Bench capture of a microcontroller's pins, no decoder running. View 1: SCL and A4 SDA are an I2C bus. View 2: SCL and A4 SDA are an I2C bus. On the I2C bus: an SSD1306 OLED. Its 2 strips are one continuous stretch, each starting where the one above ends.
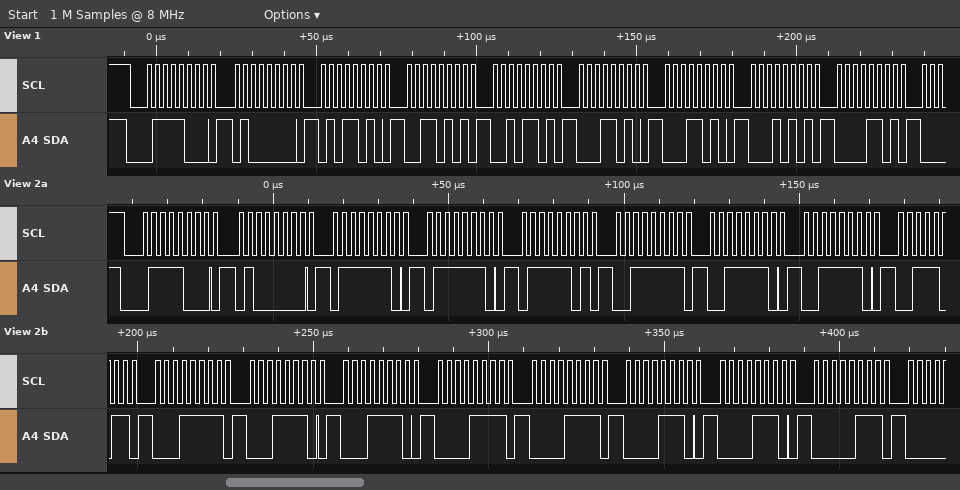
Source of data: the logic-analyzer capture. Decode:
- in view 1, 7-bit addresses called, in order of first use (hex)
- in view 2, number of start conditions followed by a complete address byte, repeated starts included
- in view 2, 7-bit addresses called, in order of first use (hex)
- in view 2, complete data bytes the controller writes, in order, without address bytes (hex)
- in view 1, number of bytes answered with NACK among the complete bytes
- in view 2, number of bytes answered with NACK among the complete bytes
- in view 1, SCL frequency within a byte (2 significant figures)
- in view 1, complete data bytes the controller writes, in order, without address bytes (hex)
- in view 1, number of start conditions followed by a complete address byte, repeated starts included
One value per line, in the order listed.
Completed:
0x3C
1
0x3C
40 7E 7E 7D 3F 3E 3E 3B 1F 1E 1E 0F 0F 0E 0E 07
0
0
400 kHz
40 5A 35 2D 1A 1A 15 0D
1
